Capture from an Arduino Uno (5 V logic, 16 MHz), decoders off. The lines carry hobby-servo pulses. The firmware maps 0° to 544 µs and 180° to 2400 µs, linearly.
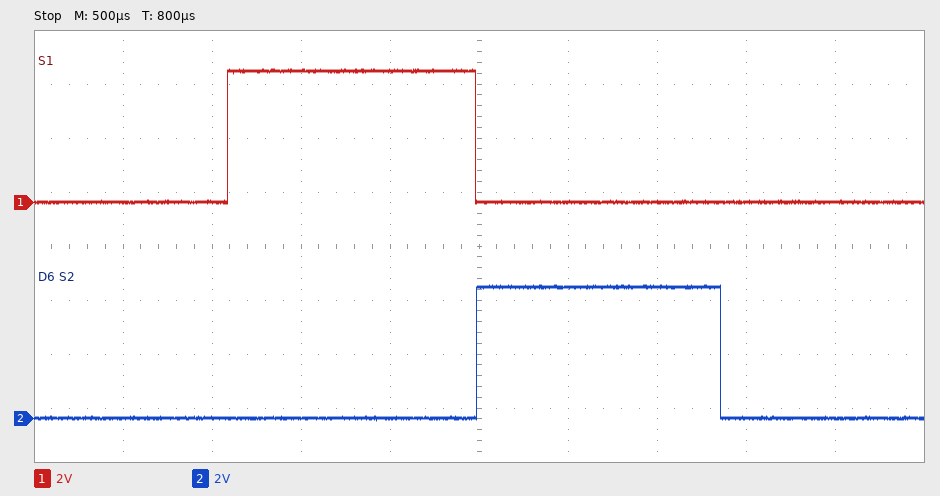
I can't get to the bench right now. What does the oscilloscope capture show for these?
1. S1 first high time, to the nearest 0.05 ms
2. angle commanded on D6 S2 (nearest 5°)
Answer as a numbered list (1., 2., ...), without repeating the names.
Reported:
1. 1.40 ms
2. 80°
